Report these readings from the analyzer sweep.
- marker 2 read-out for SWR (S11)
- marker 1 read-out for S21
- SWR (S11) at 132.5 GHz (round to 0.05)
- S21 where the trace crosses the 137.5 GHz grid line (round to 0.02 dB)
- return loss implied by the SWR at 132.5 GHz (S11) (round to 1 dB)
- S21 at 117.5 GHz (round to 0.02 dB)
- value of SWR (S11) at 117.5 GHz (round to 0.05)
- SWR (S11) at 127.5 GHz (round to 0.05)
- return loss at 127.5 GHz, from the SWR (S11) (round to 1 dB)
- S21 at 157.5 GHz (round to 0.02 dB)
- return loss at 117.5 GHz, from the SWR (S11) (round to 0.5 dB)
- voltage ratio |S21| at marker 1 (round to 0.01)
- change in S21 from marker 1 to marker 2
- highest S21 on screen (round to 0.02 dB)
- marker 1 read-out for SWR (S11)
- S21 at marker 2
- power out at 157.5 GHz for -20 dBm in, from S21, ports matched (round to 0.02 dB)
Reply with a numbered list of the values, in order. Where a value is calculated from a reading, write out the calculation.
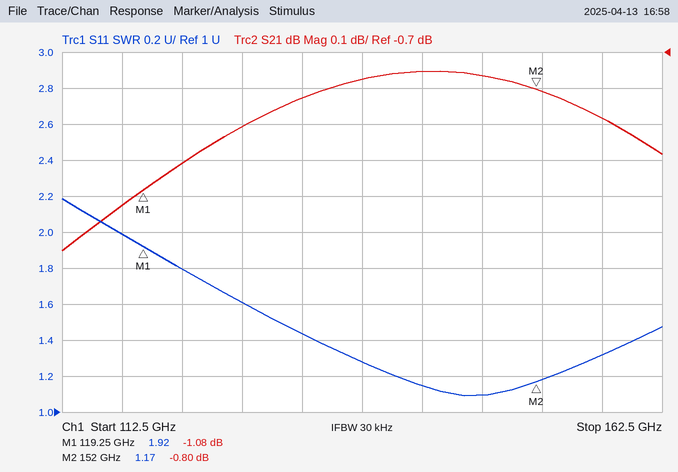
1. 1.17
2. -1.08 dB
3. 1.45
4. -0.78 dB
5. −20 log10((1.45 − 1)/(1.45 + 1)) ≈ 15 dB
6. -1.12 dB
7. 2.00
8. 1.60
9. −20 log10((1.6 − 1)/(1.6 + 1)) ≈ 13 dB
10. -0.88 dB
11. −20 log10((2 − 1)/(2 + 1)) ≈ 9.5 dB
12. 10^(-1.08/20) ≈ 0.88
13. -0.8 − (-1.08) = 0.28 dB
14. -0.76 dB
15. 1.92
16. -0.80 dB
17. -20 dBm + (-0.88 dB) = -20.88 dBm
